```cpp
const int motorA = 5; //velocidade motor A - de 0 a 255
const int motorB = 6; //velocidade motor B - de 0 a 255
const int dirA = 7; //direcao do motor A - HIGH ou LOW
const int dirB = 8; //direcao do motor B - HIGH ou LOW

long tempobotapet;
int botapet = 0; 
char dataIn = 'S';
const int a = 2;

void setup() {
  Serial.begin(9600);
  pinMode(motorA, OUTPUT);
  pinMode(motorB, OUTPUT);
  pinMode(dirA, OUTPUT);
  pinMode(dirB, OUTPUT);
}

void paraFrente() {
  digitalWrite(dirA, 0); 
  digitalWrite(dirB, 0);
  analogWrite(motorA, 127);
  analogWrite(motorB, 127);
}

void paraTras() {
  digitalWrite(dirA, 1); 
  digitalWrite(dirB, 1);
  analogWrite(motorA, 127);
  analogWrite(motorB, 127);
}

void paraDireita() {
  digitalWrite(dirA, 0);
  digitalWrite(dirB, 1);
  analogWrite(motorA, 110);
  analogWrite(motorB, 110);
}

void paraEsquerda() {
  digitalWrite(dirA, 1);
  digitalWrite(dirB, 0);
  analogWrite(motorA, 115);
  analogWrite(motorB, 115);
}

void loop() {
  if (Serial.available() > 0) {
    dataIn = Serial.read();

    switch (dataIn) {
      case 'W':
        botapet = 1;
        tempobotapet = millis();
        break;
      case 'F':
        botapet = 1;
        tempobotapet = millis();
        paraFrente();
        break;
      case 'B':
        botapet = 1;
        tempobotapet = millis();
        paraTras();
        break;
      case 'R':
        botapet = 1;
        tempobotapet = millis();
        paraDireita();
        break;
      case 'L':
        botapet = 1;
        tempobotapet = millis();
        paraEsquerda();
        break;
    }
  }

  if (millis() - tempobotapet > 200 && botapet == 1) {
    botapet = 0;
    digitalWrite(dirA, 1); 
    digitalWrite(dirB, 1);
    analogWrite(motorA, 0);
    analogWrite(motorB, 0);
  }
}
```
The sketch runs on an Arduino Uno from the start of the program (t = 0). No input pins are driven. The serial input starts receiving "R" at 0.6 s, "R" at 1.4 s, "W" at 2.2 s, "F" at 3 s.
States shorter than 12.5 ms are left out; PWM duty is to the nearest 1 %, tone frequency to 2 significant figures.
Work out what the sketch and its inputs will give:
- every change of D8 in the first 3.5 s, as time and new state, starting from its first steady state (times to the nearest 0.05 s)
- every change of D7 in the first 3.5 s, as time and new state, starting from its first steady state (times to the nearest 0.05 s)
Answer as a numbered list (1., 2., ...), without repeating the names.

1. 0 s low; 0.6 s high; 3 s low; 3.2 s high
2. 0 s low; 0.8 s high; 1.4 s low; 1.6 s high; 3 s low; 3.2 s high
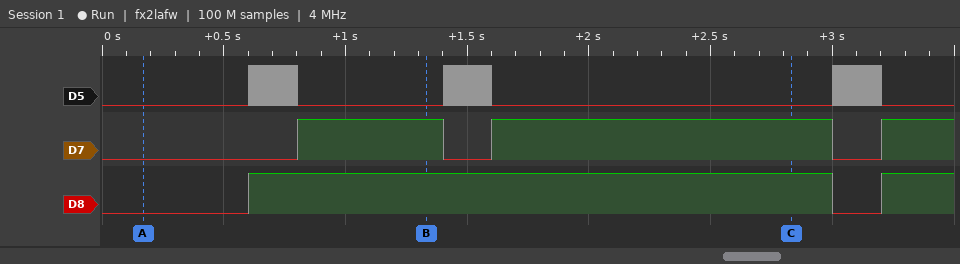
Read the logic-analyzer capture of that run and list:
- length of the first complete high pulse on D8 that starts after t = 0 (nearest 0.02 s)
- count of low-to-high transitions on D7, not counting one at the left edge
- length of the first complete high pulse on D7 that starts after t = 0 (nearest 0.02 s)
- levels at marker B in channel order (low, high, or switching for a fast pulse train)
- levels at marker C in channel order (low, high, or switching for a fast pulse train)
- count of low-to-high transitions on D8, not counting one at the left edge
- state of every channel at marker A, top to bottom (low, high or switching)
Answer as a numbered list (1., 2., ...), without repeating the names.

1. 2.40 s
2. 3
3. 0.60 s
4. D5 low, D7 high, D8 high
5. D5 low, D7 high, D8 high
6. 2
7. D5 low, D7 low, D8 low
